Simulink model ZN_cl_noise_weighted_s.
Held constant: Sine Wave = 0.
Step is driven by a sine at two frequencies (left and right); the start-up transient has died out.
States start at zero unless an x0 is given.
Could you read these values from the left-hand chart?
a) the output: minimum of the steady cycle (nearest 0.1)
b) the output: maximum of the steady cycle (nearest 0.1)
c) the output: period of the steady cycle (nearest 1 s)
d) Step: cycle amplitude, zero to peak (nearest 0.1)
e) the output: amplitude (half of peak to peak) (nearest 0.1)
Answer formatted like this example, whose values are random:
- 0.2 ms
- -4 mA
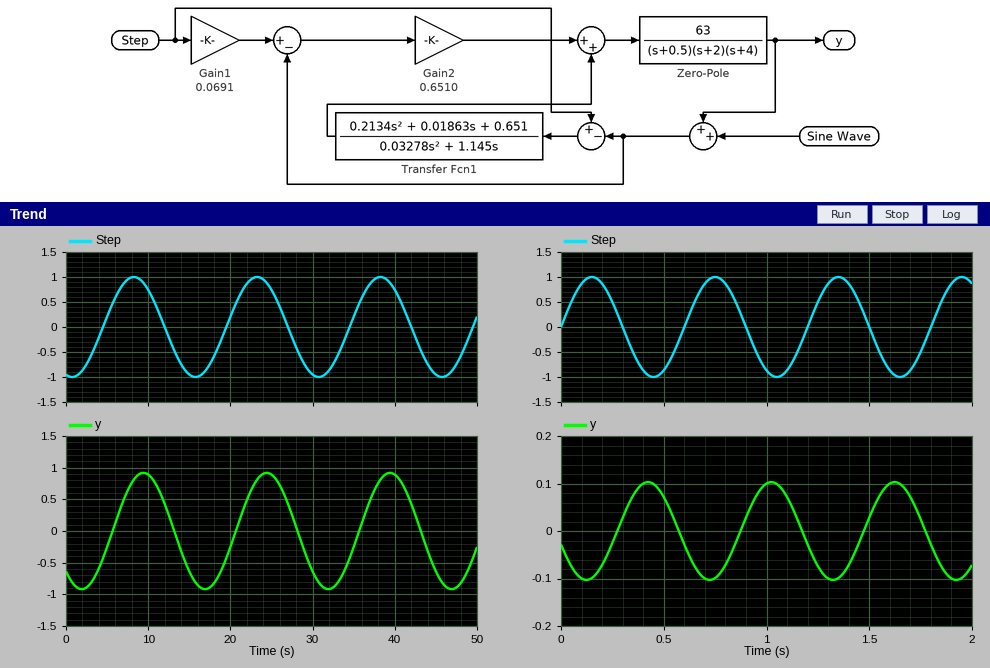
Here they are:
- -0.9
- 0.9
- 15 s
- 1.0
- 0.9
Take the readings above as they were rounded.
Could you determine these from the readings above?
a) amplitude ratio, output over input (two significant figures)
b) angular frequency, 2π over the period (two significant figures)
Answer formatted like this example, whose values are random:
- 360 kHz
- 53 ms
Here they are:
- 0.90
- 0.42 rad/s
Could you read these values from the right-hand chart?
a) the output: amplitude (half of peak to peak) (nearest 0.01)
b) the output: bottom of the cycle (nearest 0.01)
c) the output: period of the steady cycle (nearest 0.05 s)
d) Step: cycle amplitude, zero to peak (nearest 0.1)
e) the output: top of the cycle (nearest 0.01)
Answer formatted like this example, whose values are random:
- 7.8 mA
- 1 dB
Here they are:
- 0.10
- -0.10
- 0.60 s
- 1.0
- 0.10
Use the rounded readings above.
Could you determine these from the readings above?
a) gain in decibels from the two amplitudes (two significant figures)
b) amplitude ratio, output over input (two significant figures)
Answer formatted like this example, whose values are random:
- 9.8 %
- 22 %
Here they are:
- -20 dB
- 0.10
